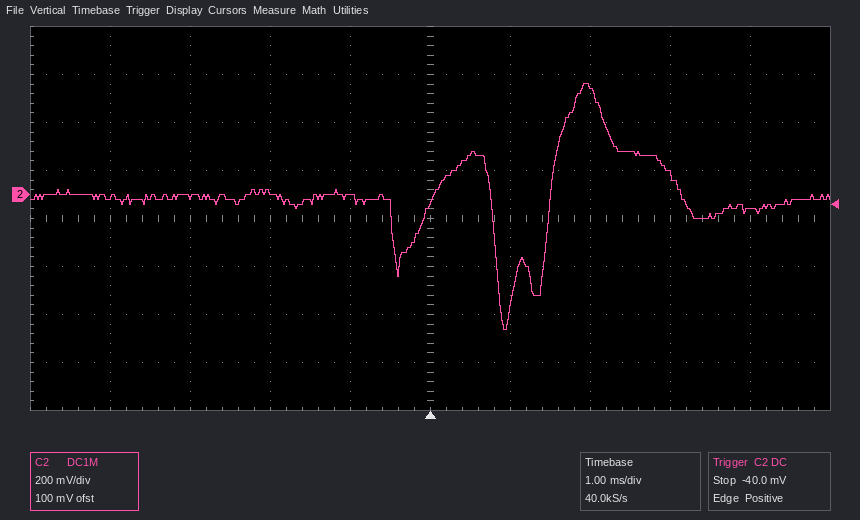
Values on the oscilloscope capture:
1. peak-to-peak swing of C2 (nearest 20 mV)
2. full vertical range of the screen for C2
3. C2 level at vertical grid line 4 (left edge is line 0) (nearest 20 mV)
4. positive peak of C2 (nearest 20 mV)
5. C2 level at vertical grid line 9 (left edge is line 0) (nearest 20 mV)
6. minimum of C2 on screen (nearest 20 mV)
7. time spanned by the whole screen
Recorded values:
1.02 V
1.6 V
0 mV
460 mV
-60 mV
-560 mV
10 ms
